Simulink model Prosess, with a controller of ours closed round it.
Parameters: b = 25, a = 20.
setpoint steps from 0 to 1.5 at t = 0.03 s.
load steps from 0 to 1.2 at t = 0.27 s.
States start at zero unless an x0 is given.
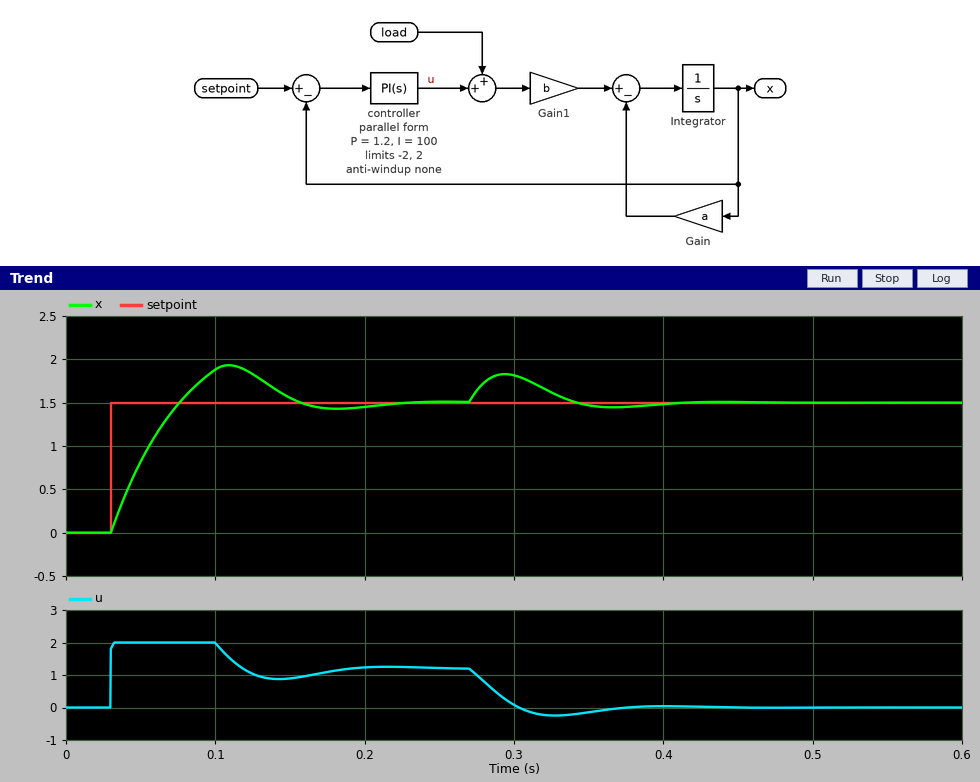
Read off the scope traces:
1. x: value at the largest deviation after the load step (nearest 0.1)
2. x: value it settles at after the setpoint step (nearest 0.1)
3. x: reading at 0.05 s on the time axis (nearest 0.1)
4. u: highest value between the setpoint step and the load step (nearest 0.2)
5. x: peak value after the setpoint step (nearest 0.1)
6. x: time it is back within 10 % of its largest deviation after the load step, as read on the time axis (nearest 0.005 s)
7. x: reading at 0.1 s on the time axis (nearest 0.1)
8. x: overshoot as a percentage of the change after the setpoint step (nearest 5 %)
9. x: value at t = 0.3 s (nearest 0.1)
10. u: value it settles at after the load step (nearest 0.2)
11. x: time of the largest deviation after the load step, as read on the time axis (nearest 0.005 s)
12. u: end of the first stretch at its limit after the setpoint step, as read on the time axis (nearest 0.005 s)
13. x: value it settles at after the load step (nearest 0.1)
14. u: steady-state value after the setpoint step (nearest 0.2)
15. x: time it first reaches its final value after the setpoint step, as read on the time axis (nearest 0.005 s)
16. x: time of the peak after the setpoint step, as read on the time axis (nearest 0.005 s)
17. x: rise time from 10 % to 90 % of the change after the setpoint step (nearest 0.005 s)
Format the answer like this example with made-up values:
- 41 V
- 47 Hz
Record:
- 1.8
- 1.5
- 0.8
- 2.0
- 1.9
- 0.390 s
- 1.9
- 30 %
- 1.8
- 0.0
- 0.295 s
- 0.100 s
- 1.5
- 1.2
- 0.075 s
- 0.110 s
- 0.035 s
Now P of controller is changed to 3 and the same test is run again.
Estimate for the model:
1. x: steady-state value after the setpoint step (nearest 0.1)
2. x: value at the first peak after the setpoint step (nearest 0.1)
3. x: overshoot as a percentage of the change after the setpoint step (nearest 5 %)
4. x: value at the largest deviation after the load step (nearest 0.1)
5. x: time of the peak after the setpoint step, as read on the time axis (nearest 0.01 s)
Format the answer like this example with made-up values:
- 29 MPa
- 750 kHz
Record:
- 1.5
- 1.8
- 20 %
- 1.7
- 0.10 s
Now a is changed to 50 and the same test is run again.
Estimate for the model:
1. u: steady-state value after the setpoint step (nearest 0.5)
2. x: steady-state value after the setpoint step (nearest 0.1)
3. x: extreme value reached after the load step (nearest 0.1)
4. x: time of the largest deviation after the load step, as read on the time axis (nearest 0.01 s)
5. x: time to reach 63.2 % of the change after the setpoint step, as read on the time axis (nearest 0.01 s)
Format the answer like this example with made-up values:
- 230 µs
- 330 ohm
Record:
- 2.0
- 1.0
- 1.6
- 0.60 s
- 0.05 s
